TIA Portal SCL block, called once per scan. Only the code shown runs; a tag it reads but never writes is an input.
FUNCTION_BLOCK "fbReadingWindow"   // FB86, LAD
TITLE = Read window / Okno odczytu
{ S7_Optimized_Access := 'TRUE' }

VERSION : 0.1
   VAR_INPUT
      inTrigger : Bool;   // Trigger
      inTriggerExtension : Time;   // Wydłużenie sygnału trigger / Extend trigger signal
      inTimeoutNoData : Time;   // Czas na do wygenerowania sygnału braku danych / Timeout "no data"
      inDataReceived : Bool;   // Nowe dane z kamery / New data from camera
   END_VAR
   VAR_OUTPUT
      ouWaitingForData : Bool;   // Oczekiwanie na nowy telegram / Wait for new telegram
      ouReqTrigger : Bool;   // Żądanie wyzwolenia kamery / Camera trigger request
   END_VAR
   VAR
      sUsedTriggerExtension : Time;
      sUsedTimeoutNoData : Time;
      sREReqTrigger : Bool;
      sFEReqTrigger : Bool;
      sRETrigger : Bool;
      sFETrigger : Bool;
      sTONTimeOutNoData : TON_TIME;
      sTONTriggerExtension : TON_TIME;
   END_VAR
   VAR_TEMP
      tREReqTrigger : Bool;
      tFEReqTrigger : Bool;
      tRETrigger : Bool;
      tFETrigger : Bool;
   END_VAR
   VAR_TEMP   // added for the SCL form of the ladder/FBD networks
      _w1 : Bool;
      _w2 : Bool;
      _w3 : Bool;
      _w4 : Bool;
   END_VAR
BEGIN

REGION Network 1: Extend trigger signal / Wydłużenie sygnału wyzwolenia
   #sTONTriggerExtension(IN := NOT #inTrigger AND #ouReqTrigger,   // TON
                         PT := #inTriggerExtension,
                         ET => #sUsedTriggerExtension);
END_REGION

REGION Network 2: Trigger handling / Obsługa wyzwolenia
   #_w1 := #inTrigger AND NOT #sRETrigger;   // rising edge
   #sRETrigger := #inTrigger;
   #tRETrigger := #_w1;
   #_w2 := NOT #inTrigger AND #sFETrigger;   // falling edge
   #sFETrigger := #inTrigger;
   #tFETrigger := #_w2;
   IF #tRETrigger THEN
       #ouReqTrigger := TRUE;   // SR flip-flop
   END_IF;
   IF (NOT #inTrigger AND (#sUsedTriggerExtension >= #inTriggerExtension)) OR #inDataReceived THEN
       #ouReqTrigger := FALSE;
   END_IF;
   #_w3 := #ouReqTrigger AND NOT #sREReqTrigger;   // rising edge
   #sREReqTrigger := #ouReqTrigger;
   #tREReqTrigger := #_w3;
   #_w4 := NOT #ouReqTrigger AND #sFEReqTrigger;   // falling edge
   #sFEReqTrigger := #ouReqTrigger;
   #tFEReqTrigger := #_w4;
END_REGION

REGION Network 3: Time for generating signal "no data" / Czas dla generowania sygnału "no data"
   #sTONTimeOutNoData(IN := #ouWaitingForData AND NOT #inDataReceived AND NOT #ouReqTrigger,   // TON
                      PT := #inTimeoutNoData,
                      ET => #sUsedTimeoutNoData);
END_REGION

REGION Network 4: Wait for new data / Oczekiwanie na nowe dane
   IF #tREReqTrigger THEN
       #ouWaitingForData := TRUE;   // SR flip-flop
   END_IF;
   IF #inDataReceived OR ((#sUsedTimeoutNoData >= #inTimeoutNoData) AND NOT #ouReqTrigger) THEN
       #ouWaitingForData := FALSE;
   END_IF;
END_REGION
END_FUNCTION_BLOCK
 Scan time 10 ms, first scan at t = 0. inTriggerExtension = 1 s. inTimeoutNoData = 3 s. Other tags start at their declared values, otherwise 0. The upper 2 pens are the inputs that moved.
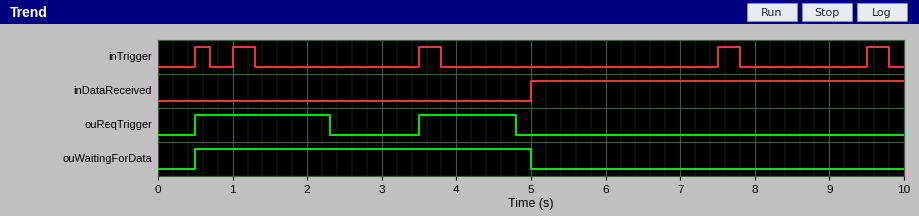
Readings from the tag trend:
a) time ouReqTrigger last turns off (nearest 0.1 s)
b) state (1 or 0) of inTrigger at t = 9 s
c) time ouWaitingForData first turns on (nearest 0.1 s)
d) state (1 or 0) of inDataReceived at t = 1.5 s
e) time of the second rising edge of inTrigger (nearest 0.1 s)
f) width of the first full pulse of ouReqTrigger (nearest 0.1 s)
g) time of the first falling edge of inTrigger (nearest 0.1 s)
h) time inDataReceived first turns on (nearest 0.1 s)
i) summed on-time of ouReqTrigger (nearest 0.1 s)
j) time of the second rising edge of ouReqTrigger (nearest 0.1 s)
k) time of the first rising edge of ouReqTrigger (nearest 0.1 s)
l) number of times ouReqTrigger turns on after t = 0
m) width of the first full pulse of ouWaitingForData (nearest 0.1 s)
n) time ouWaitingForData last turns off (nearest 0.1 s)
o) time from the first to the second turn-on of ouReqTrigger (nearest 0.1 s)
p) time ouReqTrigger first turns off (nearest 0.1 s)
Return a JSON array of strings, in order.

["4.8 s", "0", "0.5 s", "0", "1.0 s", "1.8 s", "0.7 s", "5.0 s", "3.1 s", "3.5 s", "0.5 s", "2", "4.5 s", "5.0 s", "3.0 s", "2.3 s"]
